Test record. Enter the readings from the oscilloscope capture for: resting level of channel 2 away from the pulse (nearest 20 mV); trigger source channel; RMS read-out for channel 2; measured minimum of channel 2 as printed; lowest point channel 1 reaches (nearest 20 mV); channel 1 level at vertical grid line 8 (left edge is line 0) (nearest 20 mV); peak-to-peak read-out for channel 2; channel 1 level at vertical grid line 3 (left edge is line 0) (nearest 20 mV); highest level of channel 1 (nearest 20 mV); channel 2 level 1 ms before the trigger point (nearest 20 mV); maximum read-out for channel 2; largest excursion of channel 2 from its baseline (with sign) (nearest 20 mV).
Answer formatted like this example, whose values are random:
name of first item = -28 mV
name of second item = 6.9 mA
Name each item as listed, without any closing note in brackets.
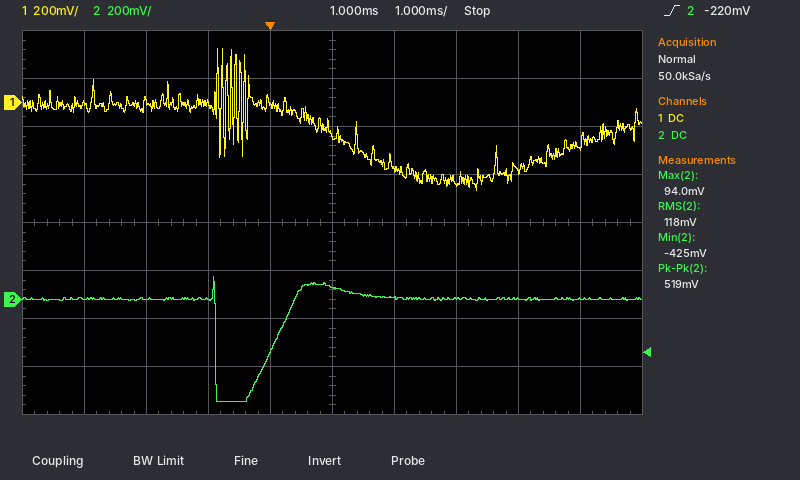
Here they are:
resting level of channel 2 away from the pulse = 0 mV
trigger source channel = channel 2
RMS read-out for channel 2 = 118 mV
measured minimum of channel 2 as printed = -425 mV
lowest point channel 1 reaches = -360 mV
channel 1 level at vertical grid line 8 (left edge is line 0) = -280 mV
peak-to-peak read-out for channel 2 = 519 mV
channel 1 level at vertical grid line 3 (left edge is line 0) = 0 mV
highest level of channel 1 = 220 mV
channel 2 level 1 ms before the trigger point = 0 mV
maximum read-out for channel 2 = 94.0 mV
largest excursion of channel 2 from its baseline (with sign) = -420 mV
